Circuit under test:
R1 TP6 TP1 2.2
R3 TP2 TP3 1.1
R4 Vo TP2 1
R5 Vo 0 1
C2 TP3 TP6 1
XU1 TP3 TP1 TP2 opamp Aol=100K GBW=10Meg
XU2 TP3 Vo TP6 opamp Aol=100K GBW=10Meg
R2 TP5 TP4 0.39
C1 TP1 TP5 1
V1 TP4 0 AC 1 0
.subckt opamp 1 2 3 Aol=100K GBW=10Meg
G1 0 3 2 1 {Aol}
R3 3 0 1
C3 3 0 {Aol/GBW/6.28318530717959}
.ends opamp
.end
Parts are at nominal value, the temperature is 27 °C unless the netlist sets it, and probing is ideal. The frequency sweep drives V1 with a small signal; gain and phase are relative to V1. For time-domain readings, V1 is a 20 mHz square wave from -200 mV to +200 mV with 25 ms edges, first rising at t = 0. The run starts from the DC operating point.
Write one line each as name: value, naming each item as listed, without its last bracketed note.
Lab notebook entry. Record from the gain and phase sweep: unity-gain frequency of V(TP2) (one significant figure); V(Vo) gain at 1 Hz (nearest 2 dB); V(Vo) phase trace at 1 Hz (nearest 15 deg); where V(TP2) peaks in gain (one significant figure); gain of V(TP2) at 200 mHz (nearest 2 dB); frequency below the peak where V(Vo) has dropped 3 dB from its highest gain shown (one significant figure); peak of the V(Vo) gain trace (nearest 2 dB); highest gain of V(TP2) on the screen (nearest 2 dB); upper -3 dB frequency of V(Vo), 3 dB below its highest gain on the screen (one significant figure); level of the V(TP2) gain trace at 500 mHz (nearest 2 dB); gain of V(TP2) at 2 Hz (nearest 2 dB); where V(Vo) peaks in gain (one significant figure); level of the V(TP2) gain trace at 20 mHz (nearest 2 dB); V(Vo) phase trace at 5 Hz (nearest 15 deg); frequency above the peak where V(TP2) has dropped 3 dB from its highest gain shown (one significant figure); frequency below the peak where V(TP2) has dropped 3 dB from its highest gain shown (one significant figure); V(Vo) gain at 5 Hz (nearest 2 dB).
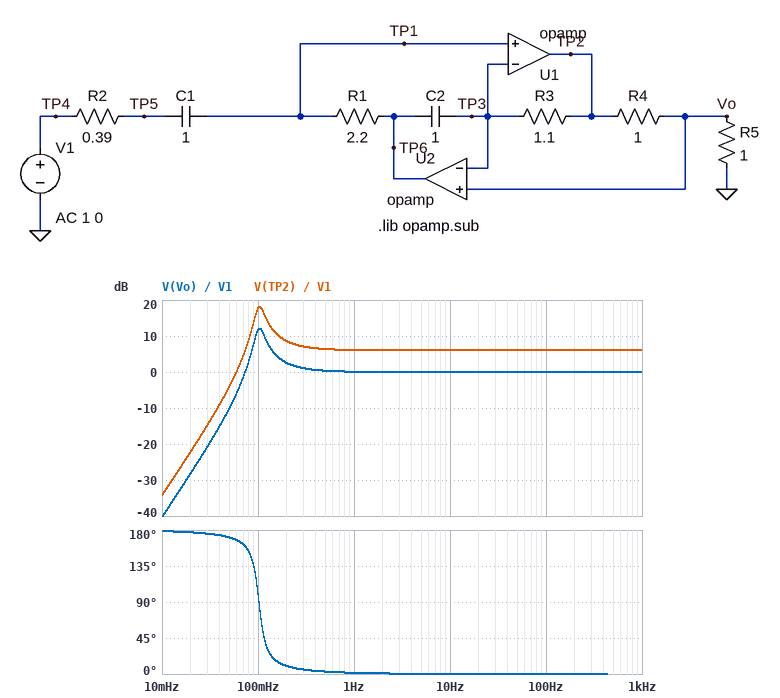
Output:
unity-gain frequency of V(TP2): 60 mHz
V(Vo) gain at 1 Hz: 0 dB
V(Vo) phase trace at 1 Hz: 0 deg
where V(TP2) peaks in gain: 100 mHz
gain of V(TP2) at 200 mHz: 8 dB
frequency below the peak where V(Vo) has dropped 3 dB from its highest gain shown: 90 mHz
peak of the V(Vo) gain trace: 12 dB
highest gain of V(TP2) on the screen: 18 dB
upper -3 dB frequency of V(Vo), 3 dB below its highest gain on the screen: 100 mHz
level of the V(TP2) gain trace at 500 mHz: 6 dB
gain of V(TP2) at 2 Hz: 6 dB
where V(Vo) peaks in gain: 100 mHz
level of the V(TP2) gain trace at 20 mHz: -22 dB
V(Vo) phase trace at 5 Hz: 0 deg
frequency above the peak where V(TP2) has dropped 3 dB from its highest gain shown: 100 mHz
frequency below the peak where V(TP2) has dropped 3 dB from its highest gain shown: 90 mHz
V(Vo) gain at 5 Hz: 0 dB
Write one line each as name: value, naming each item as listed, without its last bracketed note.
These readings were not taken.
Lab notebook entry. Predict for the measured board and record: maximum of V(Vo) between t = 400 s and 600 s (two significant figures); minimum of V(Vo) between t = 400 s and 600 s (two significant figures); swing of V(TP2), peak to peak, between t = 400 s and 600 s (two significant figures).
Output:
maximum of V(Vo) between t = 400 s and 600 s: 460 mV
minimum of V(Vo) between t = 400 s and 600 s: -460 mV
swing of V(TP2), peak to peak, between t = 400 s and 600 s: 1.8 V
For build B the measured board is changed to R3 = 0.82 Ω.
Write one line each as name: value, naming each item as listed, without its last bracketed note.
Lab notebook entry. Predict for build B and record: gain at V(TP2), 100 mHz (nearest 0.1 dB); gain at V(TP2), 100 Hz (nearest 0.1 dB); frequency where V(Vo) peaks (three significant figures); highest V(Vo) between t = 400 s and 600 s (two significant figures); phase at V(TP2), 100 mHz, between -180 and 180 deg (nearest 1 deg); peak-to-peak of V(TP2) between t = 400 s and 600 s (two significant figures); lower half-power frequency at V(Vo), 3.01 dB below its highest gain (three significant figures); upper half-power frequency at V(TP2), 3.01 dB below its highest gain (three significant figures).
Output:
gain at V(TP2), 100 mHz: 11.5 dB
gain at V(TP2), 100 Hz: 6.0 dB
frequency where V(Vo) peaks: 121 mHz
highest V(Vo) between t = 400 s and 600 s: 370 mV
phase at V(TP2), 100 mHz, between -180 and 180 deg: 140 deg
peak-to-peak of V(TP2) between t = 400 s and 600 s: 1.5 V
lower half-power frequency at V(Vo), 3.01 dB below its highest gain: 106 mHz
upper half-power frequency at V(TP2), 3.01 dB below its highest gain: 145 mHz
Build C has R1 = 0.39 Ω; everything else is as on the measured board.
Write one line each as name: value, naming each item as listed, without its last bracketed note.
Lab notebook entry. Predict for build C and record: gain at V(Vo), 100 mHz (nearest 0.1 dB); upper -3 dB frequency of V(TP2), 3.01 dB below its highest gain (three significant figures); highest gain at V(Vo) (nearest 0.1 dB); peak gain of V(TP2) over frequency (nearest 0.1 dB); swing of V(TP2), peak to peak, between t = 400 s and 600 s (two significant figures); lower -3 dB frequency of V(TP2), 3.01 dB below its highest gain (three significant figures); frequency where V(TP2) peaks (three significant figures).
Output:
gain at V(Vo), 100 mHz: -14.2 dB
upper -3 dB frequency of V(TP2), 3.01 dB below its highest gain: 482 mHz
highest gain at V(Vo): 4.9 dB
peak gain of V(TP2) over frequency: 10.9 dB
swing of V(TP2), peak to peak, between t = 400 s and 600 s: 1.6 V
lower -3 dB frequency of V(TP2), 3.01 dB below its highest gain: 206 mHz
frequency where V(TP2) peaks: 268 mHz
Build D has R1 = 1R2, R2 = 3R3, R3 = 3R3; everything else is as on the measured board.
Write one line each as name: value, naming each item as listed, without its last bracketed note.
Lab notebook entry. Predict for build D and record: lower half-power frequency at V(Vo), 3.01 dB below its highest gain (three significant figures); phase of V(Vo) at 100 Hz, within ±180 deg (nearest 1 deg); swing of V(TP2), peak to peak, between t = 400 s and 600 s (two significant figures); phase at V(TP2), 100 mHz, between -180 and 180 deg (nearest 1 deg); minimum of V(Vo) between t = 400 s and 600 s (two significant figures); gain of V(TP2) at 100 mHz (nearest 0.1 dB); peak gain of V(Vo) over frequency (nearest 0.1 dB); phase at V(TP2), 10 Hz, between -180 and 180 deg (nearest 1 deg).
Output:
lower half-power frequency at V(Vo), 3.01 dB below its highest gain: 96.1 mHz
phase of V(Vo) at 100 Hz, within ±180 deg: 0 deg
swing of V(TP2), peak to peak, between t = 400 s and 600 s: 1.6 V
phase at V(TP2), 100 mHz, between -180 and 180 deg: 75 deg
minimum of V(Vo) between t = 400 s and 600 s: -400 mV
gain of V(TP2) at 100 mHz: 3.3 dB
peak gain of V(Vo) over frequency: 0 dB
phase at V(TP2), 10 Hz, between -180 and 180 deg: 1 deg
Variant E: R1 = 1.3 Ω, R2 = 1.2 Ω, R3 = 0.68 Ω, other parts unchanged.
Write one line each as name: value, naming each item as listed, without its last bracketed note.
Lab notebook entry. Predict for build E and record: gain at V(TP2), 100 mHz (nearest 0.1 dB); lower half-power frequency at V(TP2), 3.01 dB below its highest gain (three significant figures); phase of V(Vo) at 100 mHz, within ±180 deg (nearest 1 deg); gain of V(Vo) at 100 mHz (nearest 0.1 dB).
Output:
gain at V(TP2), 100 mHz: -3.1 dB
lower half-power frequency at V(TP2), 3.01 dB below its highest gain: 157 mHz
phase of V(Vo) at 100 mHz, within ±180 deg: 131 deg
gain of V(Vo) at 100 mHz: -9.1 dB
